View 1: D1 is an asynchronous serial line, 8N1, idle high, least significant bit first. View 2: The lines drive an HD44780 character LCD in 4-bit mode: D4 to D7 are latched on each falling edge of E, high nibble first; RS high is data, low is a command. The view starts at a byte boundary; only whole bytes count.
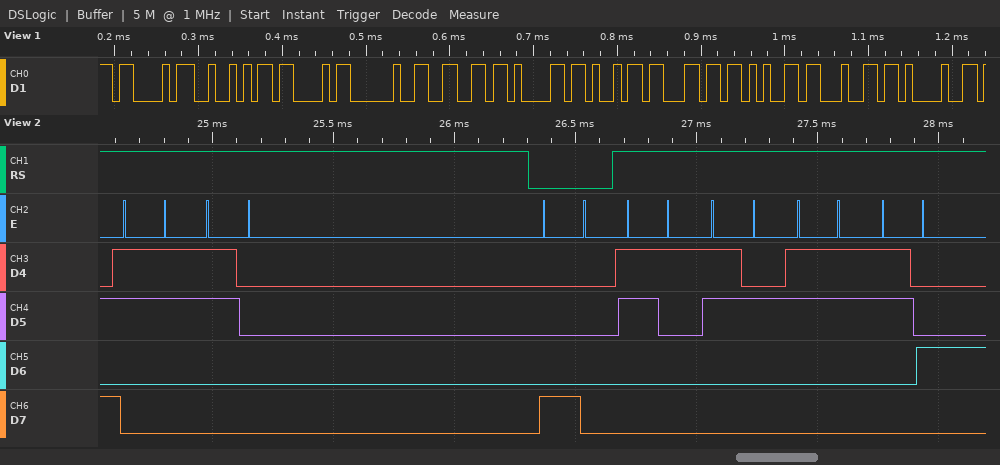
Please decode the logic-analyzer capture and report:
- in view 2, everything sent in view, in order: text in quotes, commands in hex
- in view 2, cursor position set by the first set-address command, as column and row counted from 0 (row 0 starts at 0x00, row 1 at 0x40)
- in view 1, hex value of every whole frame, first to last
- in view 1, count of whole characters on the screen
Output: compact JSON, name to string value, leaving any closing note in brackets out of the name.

{"in view 2, everything sent in view, in order: text in quotes, commands in hex": "\"30\" 0x80 \"1234\"", "in view 2, cursor position set by the first set-address command, as column and row counted from 0": "column 0, row 0", "in view 1, hex value of every whole frame, first to last": "43 52 43 20 66 61 69 6C 65 64 21", "in view 1, count of whole characters on the screen": "11"}
